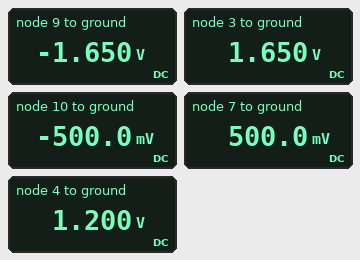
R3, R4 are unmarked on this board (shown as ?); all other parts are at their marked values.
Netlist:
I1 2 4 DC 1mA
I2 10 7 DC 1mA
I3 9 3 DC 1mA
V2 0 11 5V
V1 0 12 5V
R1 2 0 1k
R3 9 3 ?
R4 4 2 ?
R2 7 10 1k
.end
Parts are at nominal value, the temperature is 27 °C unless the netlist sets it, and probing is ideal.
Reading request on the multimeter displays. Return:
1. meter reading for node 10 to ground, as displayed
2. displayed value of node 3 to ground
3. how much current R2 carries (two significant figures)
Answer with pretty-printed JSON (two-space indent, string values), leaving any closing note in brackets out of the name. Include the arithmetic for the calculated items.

{
  "meter reading for node 10 to ground, as displayed": "-500.0 mV",
  "displayed value of node 3 to ground": "1.650 V",
  "how much current R2 carries": "(500 mV - (-500 mV)) / 1 kΩ = 1.0 mA"
}
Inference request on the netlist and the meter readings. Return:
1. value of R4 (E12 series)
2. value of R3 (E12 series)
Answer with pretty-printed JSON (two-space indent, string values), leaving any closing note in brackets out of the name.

{
  "value of R4": "1.2 kΩ",
  "value of R3": "3.3 kΩ"
}
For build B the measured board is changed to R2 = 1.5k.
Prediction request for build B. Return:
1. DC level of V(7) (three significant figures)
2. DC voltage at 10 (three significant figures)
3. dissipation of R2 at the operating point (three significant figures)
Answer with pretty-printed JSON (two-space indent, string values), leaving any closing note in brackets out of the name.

{
  "DC level of V(7)": "750 mV",
  "DC voltage at 10": "-750 mV",
  "dissipation of R2 at the operating point": "1.50 mW"
}
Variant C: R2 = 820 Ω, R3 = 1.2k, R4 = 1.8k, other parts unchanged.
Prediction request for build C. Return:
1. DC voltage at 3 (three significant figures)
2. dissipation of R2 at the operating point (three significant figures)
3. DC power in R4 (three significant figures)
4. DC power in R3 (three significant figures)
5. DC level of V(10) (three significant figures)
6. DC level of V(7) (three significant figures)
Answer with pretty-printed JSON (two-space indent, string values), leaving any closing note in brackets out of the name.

{
  "DC voltage at 3": "600 mV",
  "dissipation of R2 at the operating point": "820 µW",
  "DC power in R4": "1.80 mW",
  "DC power in R3": "1.20 mW",
  "DC level of V(10)": "-410 mV",
  "DC level of V(7)": "410 mV"
}
